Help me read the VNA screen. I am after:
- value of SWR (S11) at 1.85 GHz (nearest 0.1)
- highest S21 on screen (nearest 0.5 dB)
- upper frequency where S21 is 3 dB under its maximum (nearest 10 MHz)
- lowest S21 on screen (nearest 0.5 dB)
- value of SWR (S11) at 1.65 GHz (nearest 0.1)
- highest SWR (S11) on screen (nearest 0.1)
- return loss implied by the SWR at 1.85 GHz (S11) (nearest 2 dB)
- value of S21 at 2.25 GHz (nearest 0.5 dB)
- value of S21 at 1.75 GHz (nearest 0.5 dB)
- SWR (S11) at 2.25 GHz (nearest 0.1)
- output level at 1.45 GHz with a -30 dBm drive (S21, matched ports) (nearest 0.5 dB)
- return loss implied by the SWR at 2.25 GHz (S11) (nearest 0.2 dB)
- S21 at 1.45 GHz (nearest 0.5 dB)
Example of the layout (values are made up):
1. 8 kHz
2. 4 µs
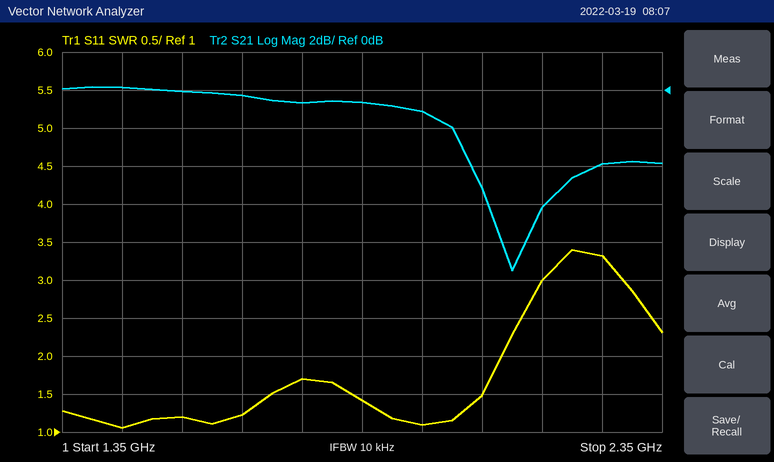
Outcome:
1. 1.4
2. 0.0 dB
3. 2.01 GHz
4. -9.5 dB
5. 1.2
6. 3.4
7. 16 dB
8. -4.0 dB
9. -0.5 dB
10. 3.3
11. -30.0 dBm
12. 5.4 dB
13. 0.0 dB
